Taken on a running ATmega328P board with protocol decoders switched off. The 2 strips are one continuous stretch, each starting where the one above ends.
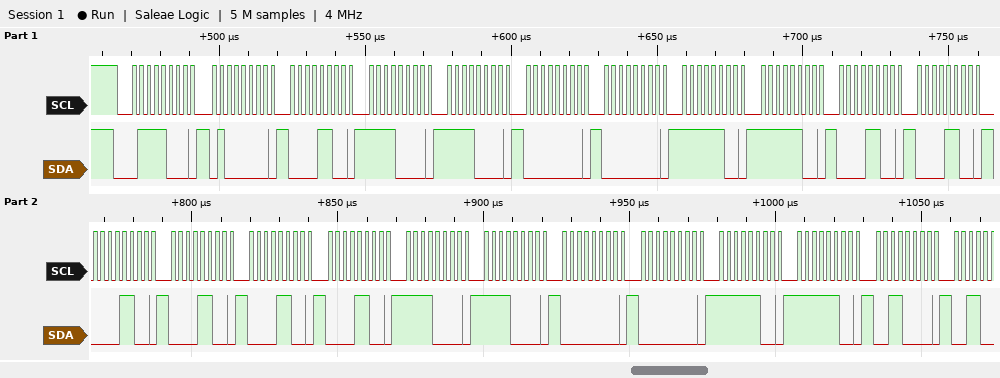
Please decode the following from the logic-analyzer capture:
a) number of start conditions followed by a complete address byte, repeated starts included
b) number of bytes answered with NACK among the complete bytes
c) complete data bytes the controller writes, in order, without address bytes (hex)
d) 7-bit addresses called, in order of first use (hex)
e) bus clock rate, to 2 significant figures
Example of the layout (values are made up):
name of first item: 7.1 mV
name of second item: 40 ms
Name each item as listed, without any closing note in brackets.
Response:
number of start conditions followed by a complete address byte, repeated starts included: 1
number of bytes answered with NACK among the complete bytes: 0
complete data bytes the controller writes, in order, without address bytes: 40 0C F0 F0 00 00 FC FC 0C 0C 0C 0C 0C 0C F0 F0 00 00 FC FC 30
7-bit addresses called, in order of first use: 0x3C
bus clock rate, to 2 significant figures: 400 kHz
